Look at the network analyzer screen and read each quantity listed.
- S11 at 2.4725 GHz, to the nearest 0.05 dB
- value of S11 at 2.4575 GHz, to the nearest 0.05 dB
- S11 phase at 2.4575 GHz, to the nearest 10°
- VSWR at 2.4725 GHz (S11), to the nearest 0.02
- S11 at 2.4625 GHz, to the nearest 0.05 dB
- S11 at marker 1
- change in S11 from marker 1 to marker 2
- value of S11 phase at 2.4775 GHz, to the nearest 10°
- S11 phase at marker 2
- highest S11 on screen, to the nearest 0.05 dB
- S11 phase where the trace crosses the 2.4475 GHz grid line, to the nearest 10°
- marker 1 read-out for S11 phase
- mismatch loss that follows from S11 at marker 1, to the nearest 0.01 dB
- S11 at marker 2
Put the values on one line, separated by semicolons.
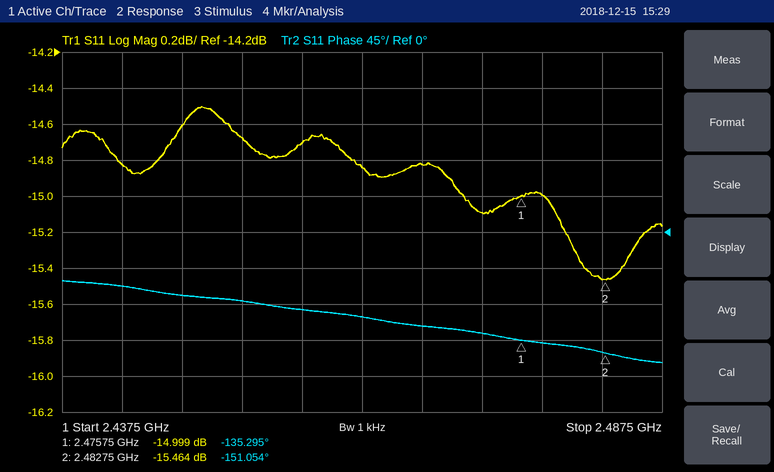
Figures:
-15.10 dB; -14.70 dB; -100°; 1.42; -14.85 dB; -14.999 dB; -0.465 dB; -140°; -151.054°; -14.50 dB; -80°; -135.295°; 0.14 dB; -15.464 dB
